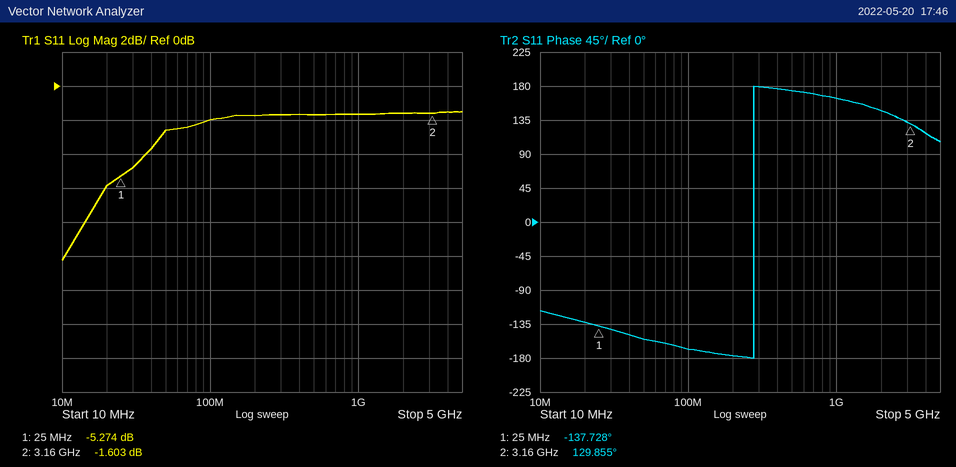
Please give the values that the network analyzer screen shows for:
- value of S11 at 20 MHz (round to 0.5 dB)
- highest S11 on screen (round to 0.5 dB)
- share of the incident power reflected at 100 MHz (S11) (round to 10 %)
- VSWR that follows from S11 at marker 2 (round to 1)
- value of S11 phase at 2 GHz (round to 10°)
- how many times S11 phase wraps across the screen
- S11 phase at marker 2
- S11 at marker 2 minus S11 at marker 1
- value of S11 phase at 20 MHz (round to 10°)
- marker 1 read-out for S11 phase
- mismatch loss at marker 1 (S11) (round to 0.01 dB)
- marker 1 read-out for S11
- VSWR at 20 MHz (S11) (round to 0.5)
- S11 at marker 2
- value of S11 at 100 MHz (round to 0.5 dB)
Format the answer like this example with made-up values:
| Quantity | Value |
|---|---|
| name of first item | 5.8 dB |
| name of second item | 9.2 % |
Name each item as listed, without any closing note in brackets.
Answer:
| Quantity | Value |
|---|---|
| value of S11 at 20 MHz | -6.0 dB |
| highest S11 on screen | -1.5 dB |
| share of the incident power reflected at 100 MHz (S11) | 60 % |
| VSWR that follows from S11 at marker 2 | 11 |
| value of S11 phase at 2 GHz | 150° |
| how many times S11 phase wraps across the screen | 1 |
| S11 phase at marker 2 | 129.855° |
| S11 at marker 2 minus S11 at marker 1 | 3.671 dB |
| value of S11 phase at 20 MHz | -130° |
| marker 1 read-out for S11 phase | -137.728° |
| mismatch loss at marker 1 (S11) | 1.53 dB |
| marker 1 read-out for S11 | -5.274 dB |
| VSWR at 20 MHz (S11) | 3.0 |
| S11 at marker 2 | -1.603 dB |
| value of S11 at 100 MHz | -2.0 dB |
